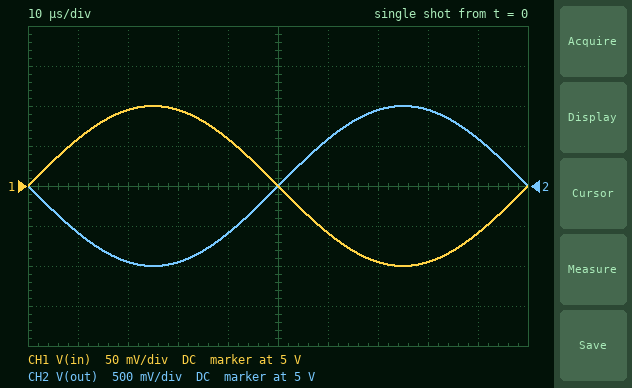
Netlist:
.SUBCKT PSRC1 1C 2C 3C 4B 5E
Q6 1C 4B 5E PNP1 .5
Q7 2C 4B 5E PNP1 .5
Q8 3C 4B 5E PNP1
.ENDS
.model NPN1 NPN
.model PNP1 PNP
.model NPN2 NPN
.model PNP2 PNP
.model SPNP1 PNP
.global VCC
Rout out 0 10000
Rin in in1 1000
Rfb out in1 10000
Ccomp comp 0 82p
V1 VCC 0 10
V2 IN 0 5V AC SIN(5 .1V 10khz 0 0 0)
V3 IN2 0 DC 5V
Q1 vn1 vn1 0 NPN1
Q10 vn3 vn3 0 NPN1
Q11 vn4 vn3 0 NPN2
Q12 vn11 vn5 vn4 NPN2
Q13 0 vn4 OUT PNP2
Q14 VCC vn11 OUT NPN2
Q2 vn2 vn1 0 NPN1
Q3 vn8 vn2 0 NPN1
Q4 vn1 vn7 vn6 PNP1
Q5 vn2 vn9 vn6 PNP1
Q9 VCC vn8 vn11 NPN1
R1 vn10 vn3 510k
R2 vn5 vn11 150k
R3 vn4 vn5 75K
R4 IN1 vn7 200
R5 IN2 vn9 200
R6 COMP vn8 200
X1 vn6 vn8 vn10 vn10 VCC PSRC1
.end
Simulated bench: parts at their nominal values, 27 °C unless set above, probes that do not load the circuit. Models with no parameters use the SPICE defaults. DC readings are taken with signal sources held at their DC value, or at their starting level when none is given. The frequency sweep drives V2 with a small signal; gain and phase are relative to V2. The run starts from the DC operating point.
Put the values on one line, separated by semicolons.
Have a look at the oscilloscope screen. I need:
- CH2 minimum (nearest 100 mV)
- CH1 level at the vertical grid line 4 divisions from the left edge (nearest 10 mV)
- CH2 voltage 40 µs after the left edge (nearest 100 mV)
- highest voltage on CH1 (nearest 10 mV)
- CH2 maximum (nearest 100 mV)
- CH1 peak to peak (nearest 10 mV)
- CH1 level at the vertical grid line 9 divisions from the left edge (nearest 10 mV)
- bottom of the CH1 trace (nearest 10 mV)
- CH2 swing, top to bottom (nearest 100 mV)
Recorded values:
4.0 V; 5.06 V; 4.4 V; 5.10 V; 6.0 V; 200 mV; 4.94 V; 4.90 V; 2.0 V
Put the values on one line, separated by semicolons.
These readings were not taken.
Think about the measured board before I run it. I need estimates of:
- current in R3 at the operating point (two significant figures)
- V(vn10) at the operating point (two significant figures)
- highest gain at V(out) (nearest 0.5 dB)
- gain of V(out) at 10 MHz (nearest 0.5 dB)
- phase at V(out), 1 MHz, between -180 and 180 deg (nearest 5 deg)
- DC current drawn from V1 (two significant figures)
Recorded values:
6.9 µA; 9.3 V; 20.0 dB; 9.5 dB; 160 deg; 1.5 mA
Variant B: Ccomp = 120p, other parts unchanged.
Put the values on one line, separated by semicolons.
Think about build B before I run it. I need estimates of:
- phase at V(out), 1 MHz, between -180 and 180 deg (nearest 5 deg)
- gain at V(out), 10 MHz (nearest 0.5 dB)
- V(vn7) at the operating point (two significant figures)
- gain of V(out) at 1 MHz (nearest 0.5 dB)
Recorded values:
155 deg; 8.5 dB; 5.0 V; 18.5 dB
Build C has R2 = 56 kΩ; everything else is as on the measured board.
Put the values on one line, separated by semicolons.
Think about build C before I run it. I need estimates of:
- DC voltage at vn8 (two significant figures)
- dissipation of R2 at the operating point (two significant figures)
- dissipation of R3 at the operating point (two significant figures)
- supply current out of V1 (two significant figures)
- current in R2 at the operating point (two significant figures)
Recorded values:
6.4 V; 4.3 µW; 5.6 µW; 550 µA; 8.7 µA
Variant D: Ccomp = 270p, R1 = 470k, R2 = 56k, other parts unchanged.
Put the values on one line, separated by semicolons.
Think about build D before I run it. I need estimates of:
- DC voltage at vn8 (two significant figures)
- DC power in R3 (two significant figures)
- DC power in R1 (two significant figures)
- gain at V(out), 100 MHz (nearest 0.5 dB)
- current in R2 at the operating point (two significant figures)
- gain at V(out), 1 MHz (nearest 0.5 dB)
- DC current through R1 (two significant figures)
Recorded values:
6.4 V; 5.7 µW; 160 µW; 7.5 dB; 8.8 µA; 15.5 dB; 18 µA
